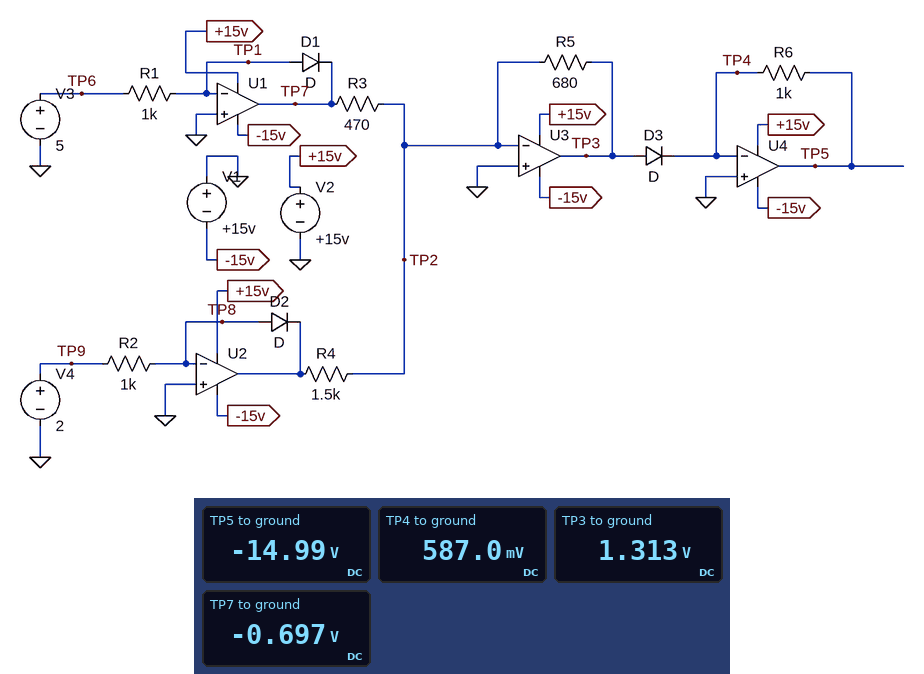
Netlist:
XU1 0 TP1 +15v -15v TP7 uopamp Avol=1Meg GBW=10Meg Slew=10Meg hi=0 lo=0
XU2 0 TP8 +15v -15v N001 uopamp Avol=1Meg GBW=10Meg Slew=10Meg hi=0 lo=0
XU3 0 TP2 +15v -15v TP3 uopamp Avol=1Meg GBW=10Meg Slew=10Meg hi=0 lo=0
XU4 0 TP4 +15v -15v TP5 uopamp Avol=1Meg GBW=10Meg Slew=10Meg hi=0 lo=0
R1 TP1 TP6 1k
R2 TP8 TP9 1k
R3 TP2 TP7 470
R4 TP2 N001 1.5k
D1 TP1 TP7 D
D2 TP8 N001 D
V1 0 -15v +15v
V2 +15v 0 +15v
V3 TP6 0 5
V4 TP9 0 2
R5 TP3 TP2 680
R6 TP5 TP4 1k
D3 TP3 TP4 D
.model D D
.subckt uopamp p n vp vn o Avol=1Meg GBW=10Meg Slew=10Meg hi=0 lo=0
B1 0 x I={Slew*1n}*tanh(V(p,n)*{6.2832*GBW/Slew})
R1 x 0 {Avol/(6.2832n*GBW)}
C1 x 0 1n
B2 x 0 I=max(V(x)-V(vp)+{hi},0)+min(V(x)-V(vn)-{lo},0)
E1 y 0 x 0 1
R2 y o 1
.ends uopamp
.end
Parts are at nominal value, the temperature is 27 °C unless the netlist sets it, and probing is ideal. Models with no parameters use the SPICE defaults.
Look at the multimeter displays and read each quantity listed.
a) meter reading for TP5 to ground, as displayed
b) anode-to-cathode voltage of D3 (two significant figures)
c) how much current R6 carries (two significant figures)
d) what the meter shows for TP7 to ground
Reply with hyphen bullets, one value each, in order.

- -14.99 V
- 730 mV
- 16 mA
- -0.697 V
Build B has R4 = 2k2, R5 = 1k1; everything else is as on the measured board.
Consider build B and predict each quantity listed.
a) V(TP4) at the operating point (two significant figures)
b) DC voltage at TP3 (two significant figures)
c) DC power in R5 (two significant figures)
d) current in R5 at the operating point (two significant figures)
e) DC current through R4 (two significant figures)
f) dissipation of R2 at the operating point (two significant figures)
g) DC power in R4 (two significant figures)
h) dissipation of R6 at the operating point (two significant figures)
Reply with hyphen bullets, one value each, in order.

- 1.2 V
- 2.0 V
- 3.5 mW
- 1.8 mA
- 310 µA
- 4.0 mW
- 210 µW
- 260 mW
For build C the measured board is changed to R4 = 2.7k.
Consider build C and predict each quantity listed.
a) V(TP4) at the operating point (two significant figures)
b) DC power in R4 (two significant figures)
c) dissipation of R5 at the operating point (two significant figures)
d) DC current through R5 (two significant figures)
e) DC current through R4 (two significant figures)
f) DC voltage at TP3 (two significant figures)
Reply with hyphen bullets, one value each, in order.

- 450 mV
- 170 µW
- 2.0 mW
- 1.7 mA
- 250 µA
- 1.2 V
